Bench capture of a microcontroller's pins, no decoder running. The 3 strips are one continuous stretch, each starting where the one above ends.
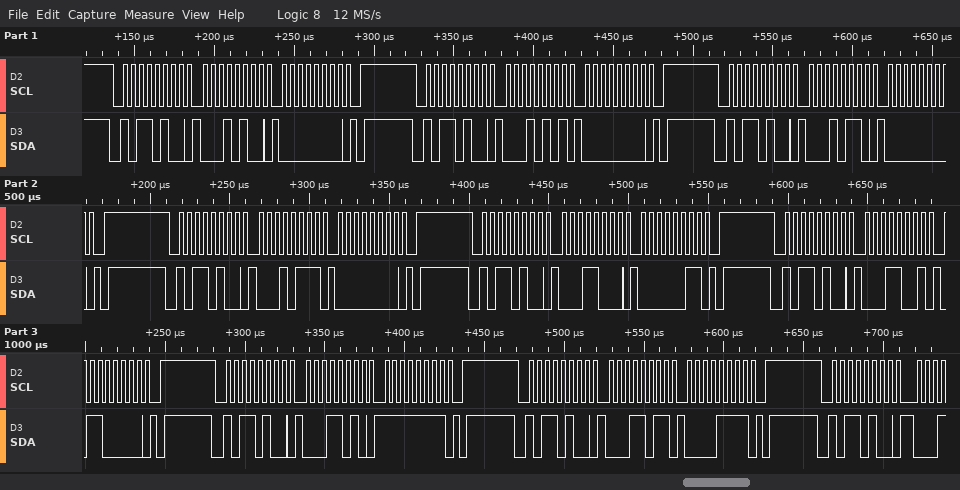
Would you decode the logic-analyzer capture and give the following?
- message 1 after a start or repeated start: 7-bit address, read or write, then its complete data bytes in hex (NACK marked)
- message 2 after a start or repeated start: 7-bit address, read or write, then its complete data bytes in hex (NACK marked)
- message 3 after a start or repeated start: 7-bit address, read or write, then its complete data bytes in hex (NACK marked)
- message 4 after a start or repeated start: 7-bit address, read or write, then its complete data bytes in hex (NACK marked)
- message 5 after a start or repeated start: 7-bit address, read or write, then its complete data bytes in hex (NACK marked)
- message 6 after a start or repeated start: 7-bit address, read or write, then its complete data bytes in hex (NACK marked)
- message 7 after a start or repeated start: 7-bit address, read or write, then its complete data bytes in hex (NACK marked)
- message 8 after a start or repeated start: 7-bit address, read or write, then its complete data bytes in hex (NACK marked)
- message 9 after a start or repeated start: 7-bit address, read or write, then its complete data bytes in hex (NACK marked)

0x5A write: 14 00
0x5A write: 15 00
0x5A write: 16 00
0x5A write: 17 00
0x5A write: 18 03
0x5A write: 19 60
0x5A write: 1A FF
0x5A write: 1B 0F
0x5A write
